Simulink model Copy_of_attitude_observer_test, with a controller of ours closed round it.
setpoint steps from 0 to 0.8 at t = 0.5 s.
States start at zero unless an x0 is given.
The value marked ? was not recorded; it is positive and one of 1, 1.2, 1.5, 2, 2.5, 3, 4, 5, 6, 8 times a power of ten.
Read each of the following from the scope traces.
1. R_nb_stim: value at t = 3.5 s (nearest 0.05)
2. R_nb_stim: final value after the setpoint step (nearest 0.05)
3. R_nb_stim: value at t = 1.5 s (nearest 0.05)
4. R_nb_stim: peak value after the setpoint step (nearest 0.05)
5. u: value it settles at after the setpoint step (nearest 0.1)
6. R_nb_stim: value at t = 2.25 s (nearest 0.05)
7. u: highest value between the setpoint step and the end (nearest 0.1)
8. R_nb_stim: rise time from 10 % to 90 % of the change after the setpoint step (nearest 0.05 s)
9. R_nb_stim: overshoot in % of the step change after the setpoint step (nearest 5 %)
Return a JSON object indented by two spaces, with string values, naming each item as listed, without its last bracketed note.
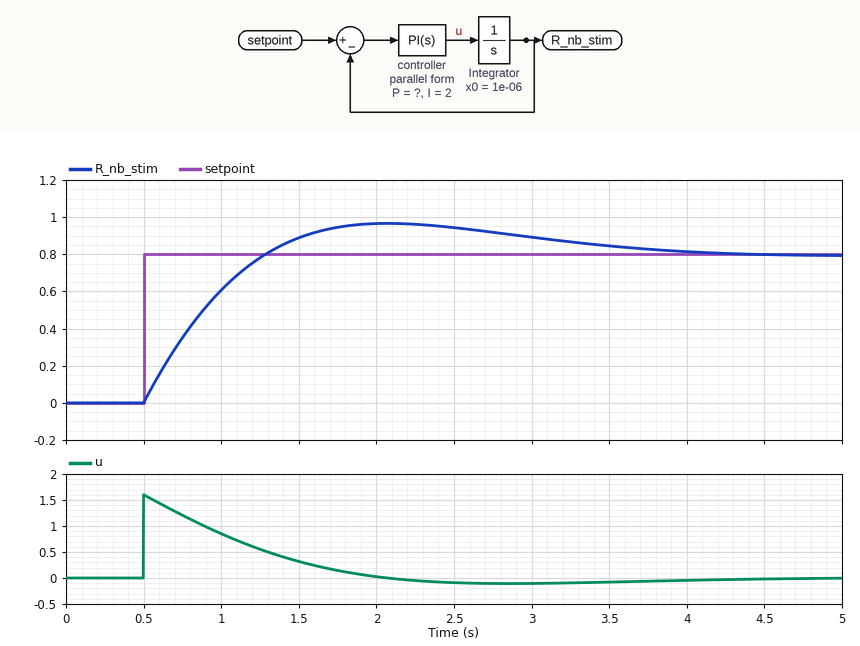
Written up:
{
  "R_nb_stim: value at t = 3.5 s": "0.85",
  "R_nb_stim: final value after the setpoint step": "0.80",
  "R_nb_stim: value at t = 1.5 s": "0.90",
  "R_nb_stim: peak value after the setpoint step": "0.95",
  "u: value it settles at after the setpoint step": "0.0",
  "R_nb_stim: value at t = 2.25 s": "0.95",
  "u: highest value between the setpoint step and the end": "1.6",
  "R_nb_stim: rise time from 10 % to 90 % of the change after the setpoint step": "0.60 s",
  "R_nb_stim: overshoot in % of the step change after the setpoint step": "20 %"
}
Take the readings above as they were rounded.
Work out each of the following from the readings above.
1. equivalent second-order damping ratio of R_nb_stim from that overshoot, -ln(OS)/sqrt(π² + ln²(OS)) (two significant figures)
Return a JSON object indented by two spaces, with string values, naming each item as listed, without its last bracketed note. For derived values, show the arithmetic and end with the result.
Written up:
{
  "equivalent second-order damping ratio of R_nb_stim from that overshoot, -ln(OS)/sqrt(π² + ln²(OS))": "ln(0.2) = -1.609; 1.609 / sqrt(9.870 + 2.590) = 0.46"
}
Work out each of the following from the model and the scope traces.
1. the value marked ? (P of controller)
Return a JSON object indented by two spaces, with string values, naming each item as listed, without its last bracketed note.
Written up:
{
  "the value marked ?": "2"
}
